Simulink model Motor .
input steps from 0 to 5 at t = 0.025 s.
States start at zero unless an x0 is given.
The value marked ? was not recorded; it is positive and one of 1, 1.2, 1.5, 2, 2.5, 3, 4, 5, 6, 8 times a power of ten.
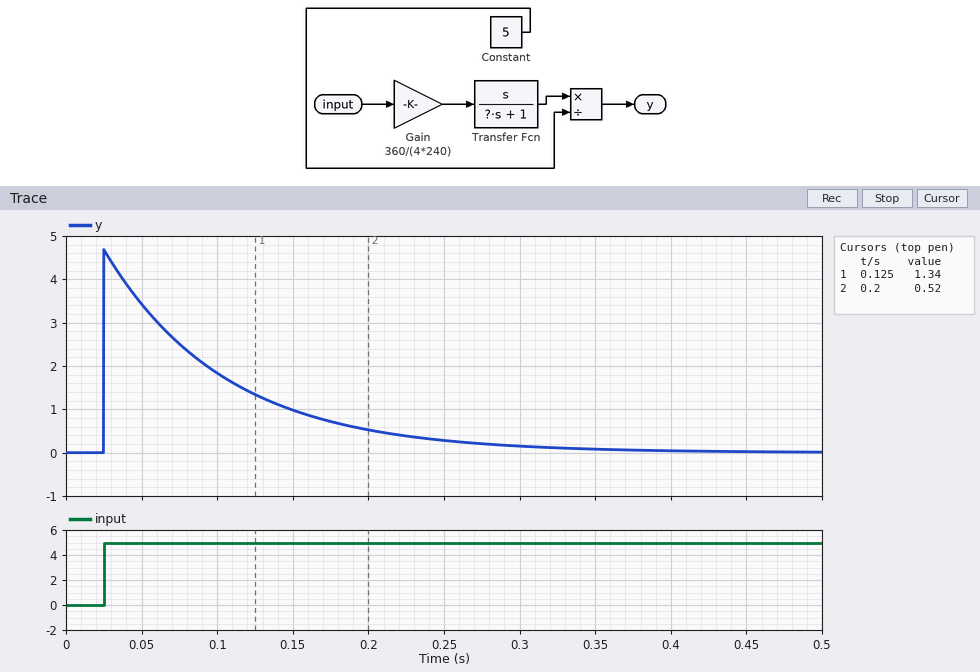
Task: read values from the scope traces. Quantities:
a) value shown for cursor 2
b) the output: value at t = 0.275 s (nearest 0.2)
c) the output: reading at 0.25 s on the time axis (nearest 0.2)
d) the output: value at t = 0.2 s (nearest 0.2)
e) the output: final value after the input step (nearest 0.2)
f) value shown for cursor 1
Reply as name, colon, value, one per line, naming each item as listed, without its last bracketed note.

value shown for cursor 2: 0.52
the output: value at t = 0.275 s: 0.2
the output: reading at 0.25 s on the time axis: 0.2
the output: value at t = 0.2 s: 0.6
the output: final value after the input step: 0.0
value shown for cursor 1: 1.34
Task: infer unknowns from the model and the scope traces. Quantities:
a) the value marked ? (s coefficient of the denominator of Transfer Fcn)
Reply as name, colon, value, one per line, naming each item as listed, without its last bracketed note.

the value marked ?: 0.08
